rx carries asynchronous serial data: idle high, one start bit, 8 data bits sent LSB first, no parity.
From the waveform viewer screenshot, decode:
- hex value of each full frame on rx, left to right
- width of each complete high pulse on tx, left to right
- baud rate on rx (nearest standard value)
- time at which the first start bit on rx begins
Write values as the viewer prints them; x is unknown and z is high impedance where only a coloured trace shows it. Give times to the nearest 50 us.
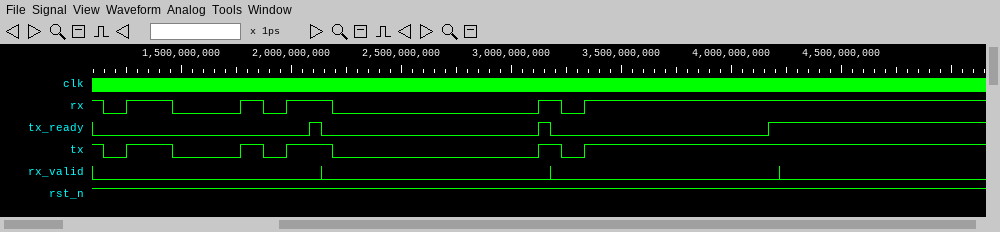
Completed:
A3, 00, FF
200 us, 100 us, 200 us, 100 us
9600 baud
1150 us
